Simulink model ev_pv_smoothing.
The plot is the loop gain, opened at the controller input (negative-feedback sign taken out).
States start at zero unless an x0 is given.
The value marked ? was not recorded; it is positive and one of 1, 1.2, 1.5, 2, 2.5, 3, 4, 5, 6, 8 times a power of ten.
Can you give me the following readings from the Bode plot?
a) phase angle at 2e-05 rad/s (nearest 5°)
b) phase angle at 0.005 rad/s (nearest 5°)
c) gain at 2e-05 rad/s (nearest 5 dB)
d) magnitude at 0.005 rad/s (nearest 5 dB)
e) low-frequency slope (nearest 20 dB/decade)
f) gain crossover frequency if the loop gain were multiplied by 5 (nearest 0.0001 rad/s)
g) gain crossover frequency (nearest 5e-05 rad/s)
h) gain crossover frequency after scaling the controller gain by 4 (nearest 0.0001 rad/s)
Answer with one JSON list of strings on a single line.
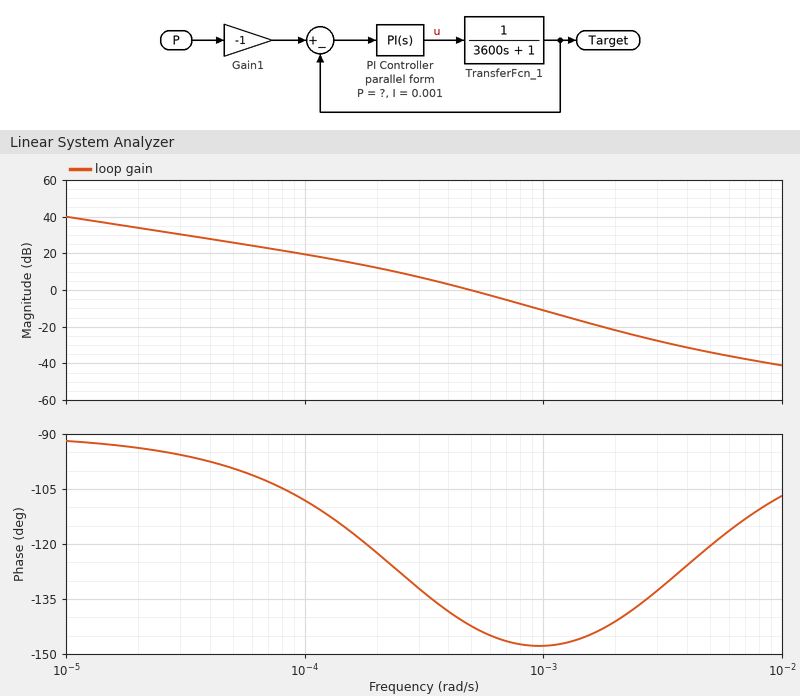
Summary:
["-95°", "-120°", "35 dB", "-35 dB", "-20 dB/decade", "0.0012 rad/s", "0.00050 rad/s", "0.0011 rad/s"]
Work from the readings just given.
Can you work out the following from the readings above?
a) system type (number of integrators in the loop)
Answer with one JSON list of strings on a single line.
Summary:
["1"]
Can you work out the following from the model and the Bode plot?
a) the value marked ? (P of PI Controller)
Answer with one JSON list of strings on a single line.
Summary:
["0.3"]
